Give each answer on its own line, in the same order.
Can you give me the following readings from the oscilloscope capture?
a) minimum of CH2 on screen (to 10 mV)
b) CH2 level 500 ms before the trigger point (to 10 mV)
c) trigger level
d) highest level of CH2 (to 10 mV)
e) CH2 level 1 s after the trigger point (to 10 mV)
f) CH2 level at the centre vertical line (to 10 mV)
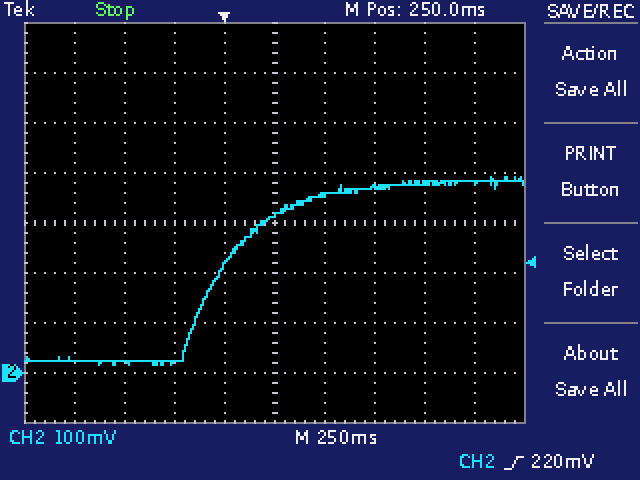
20 mV
20 mV
220 mV
390 mV
380 mV
320 mV
